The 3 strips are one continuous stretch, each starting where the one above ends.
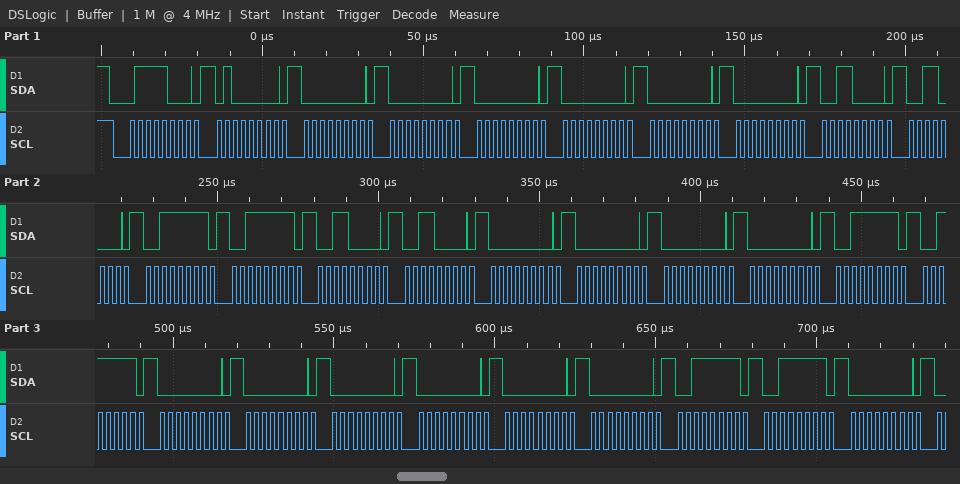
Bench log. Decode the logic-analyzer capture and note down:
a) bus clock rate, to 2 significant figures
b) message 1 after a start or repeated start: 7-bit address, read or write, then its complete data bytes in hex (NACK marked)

400 kHz
0x3C write: 40 00 00 00 00 00 00 30 30 3F 3F 30 30 00 00 00 00 3F 3F 00 00 00 00 00 00 3F 3F 00
